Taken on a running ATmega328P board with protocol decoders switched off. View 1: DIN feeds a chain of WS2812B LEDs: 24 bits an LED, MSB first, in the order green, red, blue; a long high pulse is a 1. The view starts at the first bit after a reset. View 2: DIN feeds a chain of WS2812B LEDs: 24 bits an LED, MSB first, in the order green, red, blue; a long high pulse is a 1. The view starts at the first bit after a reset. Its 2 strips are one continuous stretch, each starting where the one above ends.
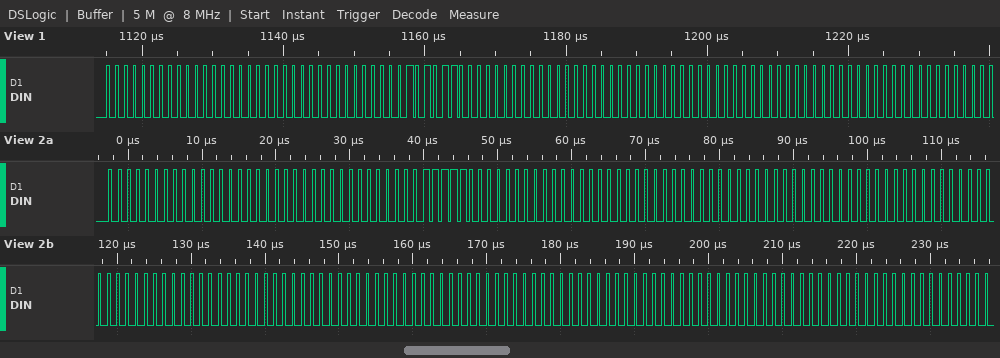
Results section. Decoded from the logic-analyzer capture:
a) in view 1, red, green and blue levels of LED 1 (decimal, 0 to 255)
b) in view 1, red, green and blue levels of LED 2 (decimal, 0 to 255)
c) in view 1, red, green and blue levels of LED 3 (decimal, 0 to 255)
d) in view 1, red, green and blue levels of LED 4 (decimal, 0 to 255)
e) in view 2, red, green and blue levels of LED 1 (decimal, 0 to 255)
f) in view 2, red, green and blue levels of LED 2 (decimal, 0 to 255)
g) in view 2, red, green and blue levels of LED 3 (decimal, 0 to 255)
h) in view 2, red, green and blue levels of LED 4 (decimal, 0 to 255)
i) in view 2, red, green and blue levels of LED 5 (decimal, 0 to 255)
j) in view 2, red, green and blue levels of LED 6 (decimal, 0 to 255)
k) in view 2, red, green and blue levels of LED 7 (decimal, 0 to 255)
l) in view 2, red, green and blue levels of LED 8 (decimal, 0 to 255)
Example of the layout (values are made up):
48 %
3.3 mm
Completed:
0, 0, 0
43, 0, 0
0, 0, 0
0, 0, 0
0, 0, 0
62, 0, 0
0, 0, 0
0, 0, 0
0, 0, 0
0, 0, 0
0, 0, 0
0, 0, 0
